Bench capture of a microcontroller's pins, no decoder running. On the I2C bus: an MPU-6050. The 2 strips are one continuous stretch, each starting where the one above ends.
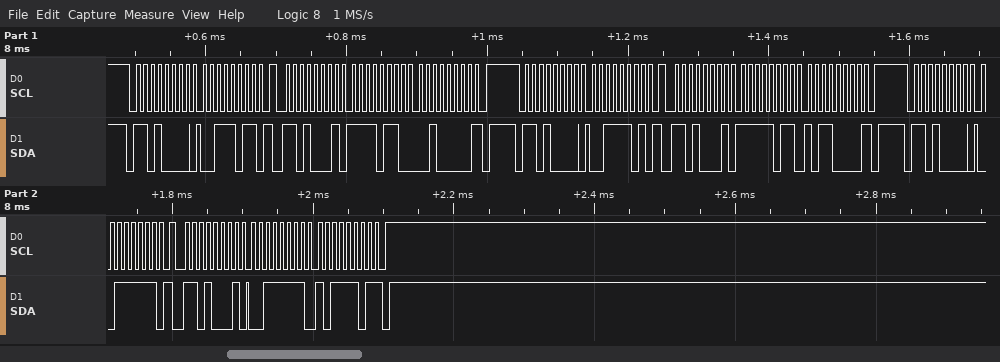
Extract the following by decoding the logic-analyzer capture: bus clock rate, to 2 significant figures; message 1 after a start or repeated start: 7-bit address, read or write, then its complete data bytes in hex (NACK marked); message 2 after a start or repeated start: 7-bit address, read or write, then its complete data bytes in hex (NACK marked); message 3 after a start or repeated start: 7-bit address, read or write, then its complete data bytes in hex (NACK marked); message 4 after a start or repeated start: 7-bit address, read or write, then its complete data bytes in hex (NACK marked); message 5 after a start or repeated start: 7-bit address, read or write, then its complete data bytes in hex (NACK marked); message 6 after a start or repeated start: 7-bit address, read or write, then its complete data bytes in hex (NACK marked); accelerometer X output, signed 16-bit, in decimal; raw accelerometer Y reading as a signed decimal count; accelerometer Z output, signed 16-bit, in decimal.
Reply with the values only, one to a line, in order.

100 kHz
0x68 write: 3B
0x68 read: F6 20 NACK
0x68 write: 3D
0x68 read: FB B0 NACK
0x68 write: 3F
0x68 read: 3F BD NACK
-2528
-1104
16317
